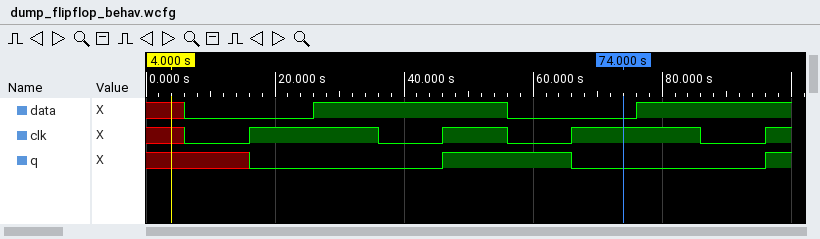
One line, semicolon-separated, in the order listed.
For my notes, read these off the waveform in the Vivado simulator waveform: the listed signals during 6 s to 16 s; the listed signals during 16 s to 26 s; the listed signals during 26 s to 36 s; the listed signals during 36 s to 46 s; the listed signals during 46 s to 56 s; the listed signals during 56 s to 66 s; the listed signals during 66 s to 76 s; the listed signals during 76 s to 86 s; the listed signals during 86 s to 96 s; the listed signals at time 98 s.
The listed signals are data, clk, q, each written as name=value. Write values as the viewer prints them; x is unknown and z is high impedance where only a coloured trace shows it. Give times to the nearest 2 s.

data=0, clk=0, q=x; data=0, clk=1, q=0; data=1, clk=1, q=0; data=1, clk=0, q=0; data=1, clk=1, q=1; data=0, clk=0, q=1; data=0, clk=1, q=0; data=1, clk=1, q=0; data=1, clk=0, q=0; data=1, clk=1, q=1
